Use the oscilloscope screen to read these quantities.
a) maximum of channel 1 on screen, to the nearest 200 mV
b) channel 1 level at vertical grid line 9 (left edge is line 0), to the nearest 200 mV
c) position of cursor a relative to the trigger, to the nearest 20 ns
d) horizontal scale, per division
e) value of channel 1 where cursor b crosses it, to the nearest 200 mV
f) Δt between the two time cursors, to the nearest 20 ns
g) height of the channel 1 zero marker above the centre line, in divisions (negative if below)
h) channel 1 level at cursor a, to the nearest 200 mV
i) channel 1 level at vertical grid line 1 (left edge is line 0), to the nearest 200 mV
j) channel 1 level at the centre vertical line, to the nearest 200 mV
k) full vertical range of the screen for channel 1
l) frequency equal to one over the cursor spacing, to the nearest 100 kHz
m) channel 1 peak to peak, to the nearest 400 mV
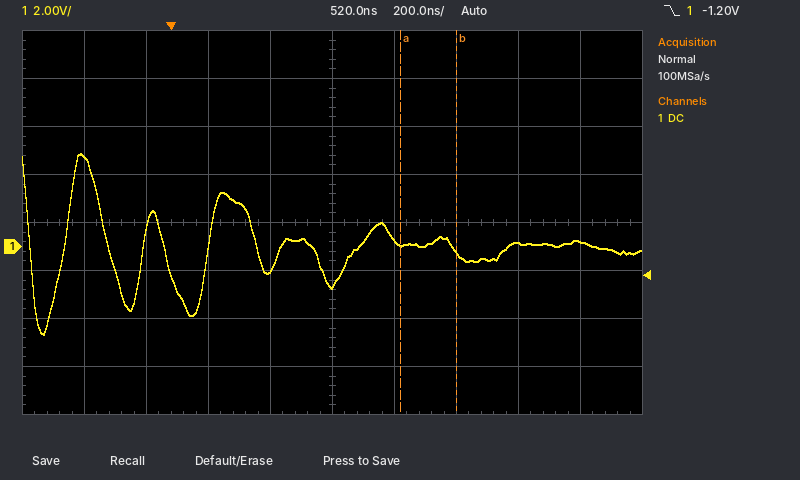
3.8 V
200 mV
+740 ns
200 ns
-200 mV
180 ns
-0.5 div
0.0 V
3.8 V
-1.6 V
16 V
5.6 MHz
7.6 V
